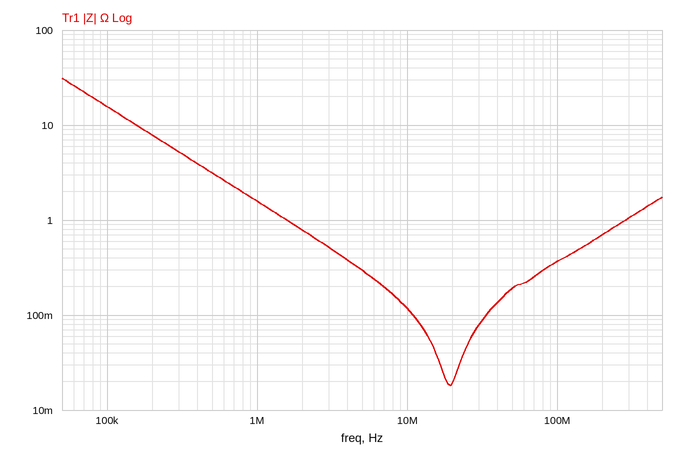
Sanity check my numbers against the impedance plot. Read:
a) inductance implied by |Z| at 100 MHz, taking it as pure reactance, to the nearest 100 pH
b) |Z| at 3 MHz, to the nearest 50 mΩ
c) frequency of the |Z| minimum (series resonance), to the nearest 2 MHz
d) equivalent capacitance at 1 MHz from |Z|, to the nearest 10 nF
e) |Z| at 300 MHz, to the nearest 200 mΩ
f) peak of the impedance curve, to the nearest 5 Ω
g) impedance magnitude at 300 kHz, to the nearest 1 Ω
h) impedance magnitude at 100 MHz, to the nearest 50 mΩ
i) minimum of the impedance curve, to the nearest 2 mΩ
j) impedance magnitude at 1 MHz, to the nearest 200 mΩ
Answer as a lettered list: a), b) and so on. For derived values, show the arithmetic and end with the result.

a) L = 350 mΩ/(2π × 100 MHz) ≈ 557 pH, so 600 pH to the nearest 100 pH
b) 500 mΩ
c) 20 MHz
d) C = 1/(2π × 1 MHz × 1.6 Ω) ≈ 100 nF
e) 1.0 Ω
f) 30 Ω
g) 5 Ω
h) 350 mΩ
i) 18 mΩ
j) 1.6 Ω
